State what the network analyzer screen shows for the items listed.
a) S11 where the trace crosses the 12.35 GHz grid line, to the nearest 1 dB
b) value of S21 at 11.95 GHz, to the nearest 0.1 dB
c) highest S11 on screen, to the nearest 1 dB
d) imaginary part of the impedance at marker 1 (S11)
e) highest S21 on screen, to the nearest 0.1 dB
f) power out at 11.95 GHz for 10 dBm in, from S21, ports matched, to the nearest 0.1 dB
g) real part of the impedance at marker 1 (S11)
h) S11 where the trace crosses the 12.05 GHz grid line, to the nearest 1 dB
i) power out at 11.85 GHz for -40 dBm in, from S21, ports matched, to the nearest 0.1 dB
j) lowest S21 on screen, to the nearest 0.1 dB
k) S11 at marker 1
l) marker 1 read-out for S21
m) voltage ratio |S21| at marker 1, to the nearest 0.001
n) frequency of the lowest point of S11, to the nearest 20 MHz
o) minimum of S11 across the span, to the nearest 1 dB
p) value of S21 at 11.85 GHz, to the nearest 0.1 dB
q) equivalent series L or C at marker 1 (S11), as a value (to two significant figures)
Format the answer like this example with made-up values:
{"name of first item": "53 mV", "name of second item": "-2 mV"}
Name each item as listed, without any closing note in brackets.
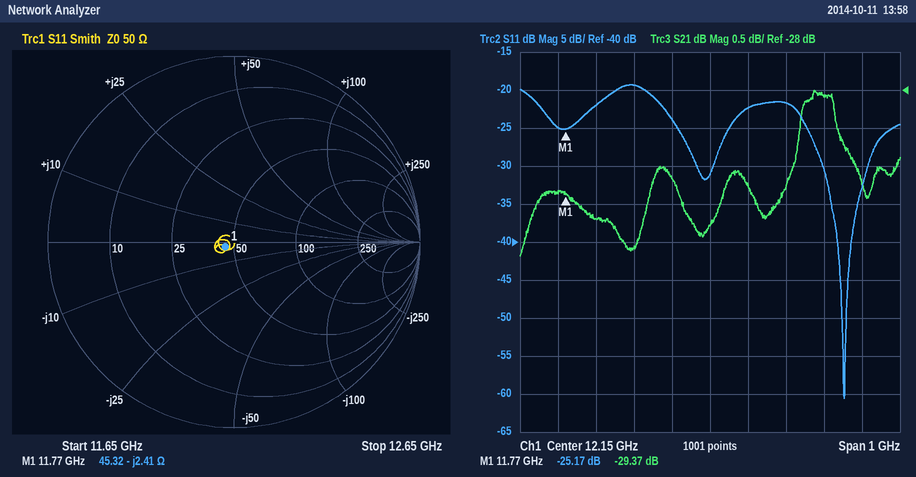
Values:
{"S11 where the trace crosses the 12.35 GHz grid line, to the nearest 1 dB": "-22 dB", "value of S21 at 11.95 GHz, to the nearest 0.1 dB": "-30.1 dB", "highest S11 on screen, to the nearest 1 dB": "-19 dB", "imaginary part of the impedance at marker 1": "-2.41 Ω", "highest S21 on screen, to the nearest 0.1 dB": "-28.0 dB", "power out at 11.95 GHz for 10 dBm in, from S21, ports matched, to the nearest 0.1 dB": "-20.1 dBm", "real part of the impedance at marker 1": "45.32 Ω", "S11 where the trace crosses the 12.05 GHz grid line, to the nearest 1 dB": "-24 dB", "power out at 11.85 GHz for -40 dBm in, from S21, ports matched, to the nearest 0.1 dB": "-69.7 dBm", "lowest S21 on screen, to the nearest 0.1 dB": "-30.2 dB", "S11 at marker 1": "-25.17 dB", "marker 1 read-out for S21": "-29.37 dB", "voltage ratio |S21| at marker 1, to the nearest 0.001": "0.034", "frequency of the lowest point of S11, to the nearest 20 MHz": "12.50 GHz", "minimum of S11 across the span, to the nearest 1 dB": "-61 dB", "value of S21 at 11.85 GHz, to the nearest 0.1 dB": "-29.7 dB", "equivalent series L or C at marker 1 (S11), as a value": "5.6 pF"}
